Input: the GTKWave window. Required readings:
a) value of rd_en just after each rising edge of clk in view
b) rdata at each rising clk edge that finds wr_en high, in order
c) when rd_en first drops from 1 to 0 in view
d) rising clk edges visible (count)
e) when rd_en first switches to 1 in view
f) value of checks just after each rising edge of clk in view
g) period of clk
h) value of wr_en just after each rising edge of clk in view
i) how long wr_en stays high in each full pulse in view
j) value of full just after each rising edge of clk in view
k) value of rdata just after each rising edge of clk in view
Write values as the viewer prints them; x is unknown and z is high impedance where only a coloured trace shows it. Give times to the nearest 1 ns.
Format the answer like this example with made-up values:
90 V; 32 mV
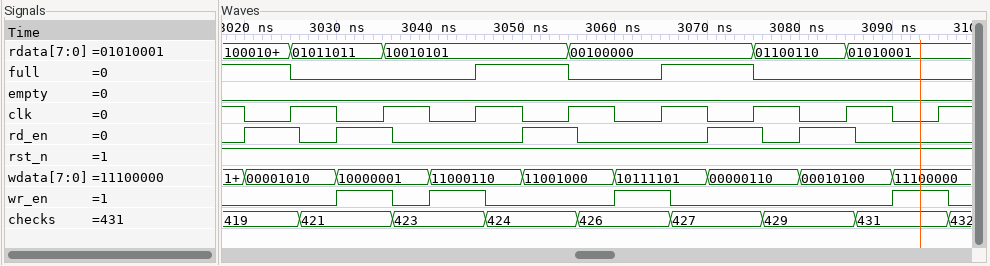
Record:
1 1 0 1 0 1 1 0; 01011011, 10010101, 00100000, 01010001; 3026 ns; 8; 3020 ns; 419, 421, 423, 424, 426, 427, 429, 431; 10 ns; 0 1 1 0 1 0 0 1; 6 ns, 6 ns, 6 ns, 6 ns; 0 0 1 0 1 0 0 0; 01011011, 10010101, 10010101, 00100000, 00100000, 01100110, 01010001, 01010001
